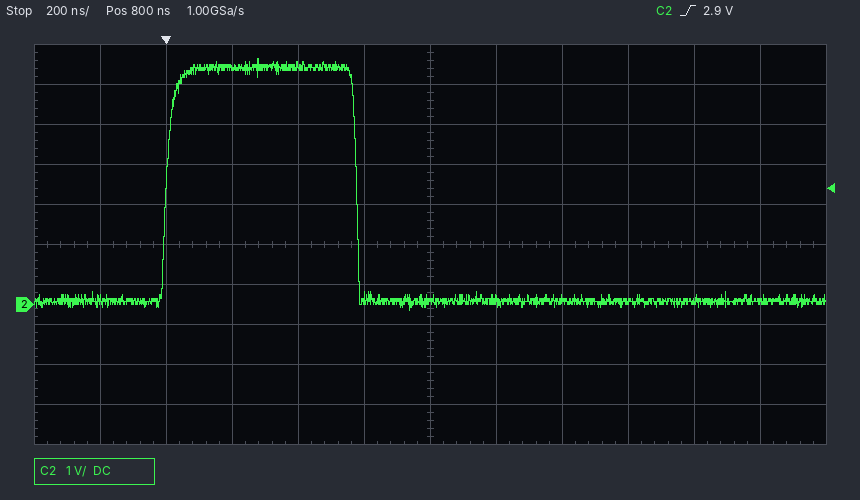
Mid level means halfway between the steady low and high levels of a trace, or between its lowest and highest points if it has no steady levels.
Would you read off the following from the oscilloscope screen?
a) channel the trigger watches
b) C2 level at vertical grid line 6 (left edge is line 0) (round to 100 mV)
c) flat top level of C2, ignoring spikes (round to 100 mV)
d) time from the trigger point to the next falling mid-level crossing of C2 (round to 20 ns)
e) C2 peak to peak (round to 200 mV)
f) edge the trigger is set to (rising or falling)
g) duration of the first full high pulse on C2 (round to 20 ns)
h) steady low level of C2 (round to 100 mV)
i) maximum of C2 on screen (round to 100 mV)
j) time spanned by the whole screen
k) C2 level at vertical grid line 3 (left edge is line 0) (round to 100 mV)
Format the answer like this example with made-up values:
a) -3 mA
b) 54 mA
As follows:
a) C2
b) 100 mV
c) 5.9 V
d) 580 ns
e) 6.4 V
f) rising
g) 580 ns
h) 100 mV
i) 6.2 V
j) 2.4 µs
k) 5.9 V
